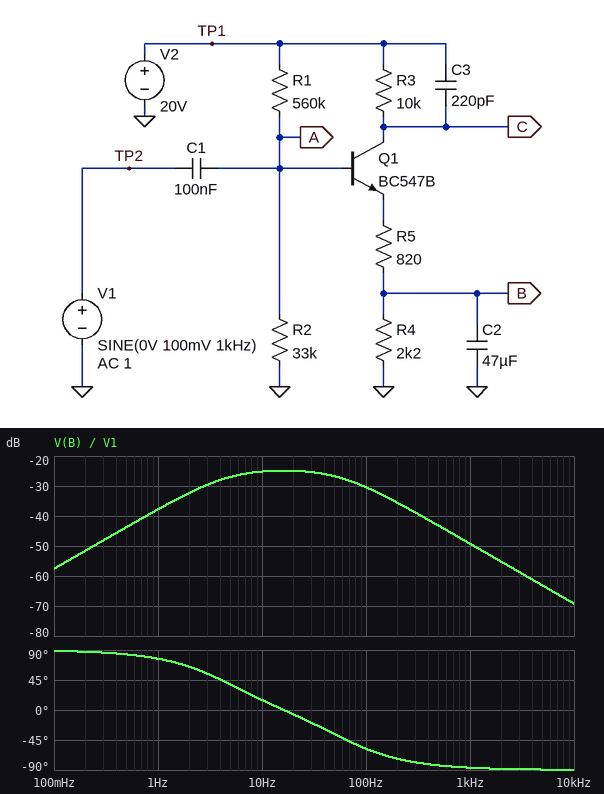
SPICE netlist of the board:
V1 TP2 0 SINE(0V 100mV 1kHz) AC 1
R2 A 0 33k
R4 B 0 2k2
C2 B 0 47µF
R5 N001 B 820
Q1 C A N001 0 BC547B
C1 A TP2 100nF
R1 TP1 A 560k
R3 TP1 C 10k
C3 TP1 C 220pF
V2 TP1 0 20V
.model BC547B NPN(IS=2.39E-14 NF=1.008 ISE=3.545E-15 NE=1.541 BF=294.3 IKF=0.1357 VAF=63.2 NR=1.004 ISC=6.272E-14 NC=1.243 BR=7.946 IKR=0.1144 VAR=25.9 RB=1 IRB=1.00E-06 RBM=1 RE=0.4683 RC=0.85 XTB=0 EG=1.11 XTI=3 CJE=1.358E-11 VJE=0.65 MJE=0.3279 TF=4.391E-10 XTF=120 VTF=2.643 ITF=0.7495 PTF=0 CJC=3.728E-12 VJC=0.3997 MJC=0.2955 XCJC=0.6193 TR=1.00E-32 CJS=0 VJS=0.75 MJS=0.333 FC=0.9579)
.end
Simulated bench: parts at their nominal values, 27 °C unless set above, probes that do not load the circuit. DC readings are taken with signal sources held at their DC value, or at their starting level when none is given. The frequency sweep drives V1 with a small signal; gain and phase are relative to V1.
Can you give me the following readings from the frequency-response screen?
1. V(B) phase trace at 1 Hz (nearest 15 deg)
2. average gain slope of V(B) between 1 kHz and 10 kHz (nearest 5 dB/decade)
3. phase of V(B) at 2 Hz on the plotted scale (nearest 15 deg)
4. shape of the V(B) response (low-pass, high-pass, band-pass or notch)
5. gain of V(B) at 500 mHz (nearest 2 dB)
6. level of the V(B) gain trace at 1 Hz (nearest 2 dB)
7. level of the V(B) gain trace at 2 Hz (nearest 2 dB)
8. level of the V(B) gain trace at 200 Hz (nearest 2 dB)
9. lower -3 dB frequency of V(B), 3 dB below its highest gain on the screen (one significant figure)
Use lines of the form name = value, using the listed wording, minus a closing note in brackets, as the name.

V(B) phase trace at 1 Hz = 75 deg
average gain slope of V(B) between 1 kHz and 10 kHz = -20 dB/decade
phase of V(B) at 2 Hz on the plotted scale = 60 deg
shape of the V(B) response = band-pass
gain of V(B) at 500 mHz = -44 dB
level of the V(B) gain trace at 1 Hz = -38 dB
level of the V(B) gain trace at 2 Hz = -32 dB
level of the V(B) gain trace at 200 Hz = -36 dB
lower -3 dB frequency of V(B), 3 dB below its highest gain on the screen = 4 Hz
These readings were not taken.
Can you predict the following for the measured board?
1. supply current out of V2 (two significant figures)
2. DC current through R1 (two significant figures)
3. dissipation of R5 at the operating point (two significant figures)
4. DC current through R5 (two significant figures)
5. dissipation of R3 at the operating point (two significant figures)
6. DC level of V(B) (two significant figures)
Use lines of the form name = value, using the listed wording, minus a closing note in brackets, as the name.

supply current out of V2 = 200 µA
DC current through R1 = 34 µA
dissipation of R5 at the operating point = 24 µW
DC current through R5 = 170 µA
dissipation of R3 at the operating point = 290 µW
DC level of V(B) = 370 mV
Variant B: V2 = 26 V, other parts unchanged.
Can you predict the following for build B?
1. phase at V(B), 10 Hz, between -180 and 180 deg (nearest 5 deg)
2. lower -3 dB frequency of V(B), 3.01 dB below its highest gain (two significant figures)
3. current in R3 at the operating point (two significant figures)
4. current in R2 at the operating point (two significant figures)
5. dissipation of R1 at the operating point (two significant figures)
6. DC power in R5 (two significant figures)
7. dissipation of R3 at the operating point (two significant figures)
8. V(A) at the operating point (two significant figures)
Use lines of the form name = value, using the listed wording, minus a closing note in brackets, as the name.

phase at V(B), 10 Hz, between -180 and 180 deg = 15 deg
lower -3 dB frequency of V(B), 3.01 dB below its highest gain = 4.2 Hz
current in R3 at the operating point = 270 µA
current in R2 at the operating point = 43 µA
dissipation of R1 at the operating point = 1.1 mW
DC power in R5 = 62 µW
dissipation of R3 at the operating point = 750 µW
V(A) at the operating point = 1.4 V
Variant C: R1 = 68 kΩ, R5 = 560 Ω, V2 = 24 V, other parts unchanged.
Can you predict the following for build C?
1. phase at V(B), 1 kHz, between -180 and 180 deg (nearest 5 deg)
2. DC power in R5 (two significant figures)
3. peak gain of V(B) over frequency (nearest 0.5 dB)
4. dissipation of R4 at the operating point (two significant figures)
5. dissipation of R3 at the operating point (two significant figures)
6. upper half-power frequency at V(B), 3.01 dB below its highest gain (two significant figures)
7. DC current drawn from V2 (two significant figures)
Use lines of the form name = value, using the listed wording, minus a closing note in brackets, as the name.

phase at V(B), 1 kHz, between -180 and 180 deg = -20 deg
DC power in R5 = 2.1 mW
peak gain of V(B) over frequency = -54.0 dB
dissipation of R4 at the operating point = 8.3 mW
dissipation of R3 at the operating point = 35 mW
upper half-power frequency at V(B), 3.01 dB below its highest gain = 2.6 kHz
DC current drawn from V2 = 2.1 mA
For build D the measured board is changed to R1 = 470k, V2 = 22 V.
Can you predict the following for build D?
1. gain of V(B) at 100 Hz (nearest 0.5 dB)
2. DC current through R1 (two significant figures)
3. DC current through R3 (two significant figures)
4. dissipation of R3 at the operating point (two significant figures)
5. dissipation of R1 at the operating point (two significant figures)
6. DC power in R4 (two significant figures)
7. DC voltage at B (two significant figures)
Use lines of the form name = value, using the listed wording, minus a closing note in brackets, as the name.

gain of V(B) at 100 Hz = -30.0 dB
DC current through R1 = 44 µA
DC current through R3 = 270 µA
dissipation of R3 at the operating point = 740 µW
dissipation of R1 at the operating point = 900 µW
DC power in R4 = 160 µW
DC voltage at B = 600 mV
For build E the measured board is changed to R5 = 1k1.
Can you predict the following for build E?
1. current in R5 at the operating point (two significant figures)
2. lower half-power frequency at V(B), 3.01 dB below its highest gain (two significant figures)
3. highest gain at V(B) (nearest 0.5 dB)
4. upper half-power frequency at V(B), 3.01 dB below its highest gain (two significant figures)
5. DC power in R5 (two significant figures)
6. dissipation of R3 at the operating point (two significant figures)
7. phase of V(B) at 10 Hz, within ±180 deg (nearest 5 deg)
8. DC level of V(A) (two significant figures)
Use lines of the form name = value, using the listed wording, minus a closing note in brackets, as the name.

current in R5 at the operating point = 160 µA
lower half-power frequency at V(B), 3.01 dB below its highest gain = 3.5 Hz
highest gain at V(B) = -27.0 dB
upper half-power frequency at V(B), 3.01 dB below its highest gain = 62 Hz
DC power in R5 = 27 µW
dissipation of R3 at the operating point = 240 µW
phase of V(B) at 10 Hz, within ±180 deg = 10 deg
DC level of V(A) = 1.1 V
